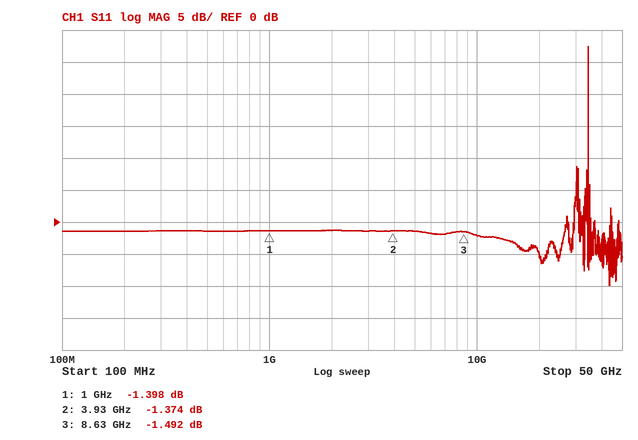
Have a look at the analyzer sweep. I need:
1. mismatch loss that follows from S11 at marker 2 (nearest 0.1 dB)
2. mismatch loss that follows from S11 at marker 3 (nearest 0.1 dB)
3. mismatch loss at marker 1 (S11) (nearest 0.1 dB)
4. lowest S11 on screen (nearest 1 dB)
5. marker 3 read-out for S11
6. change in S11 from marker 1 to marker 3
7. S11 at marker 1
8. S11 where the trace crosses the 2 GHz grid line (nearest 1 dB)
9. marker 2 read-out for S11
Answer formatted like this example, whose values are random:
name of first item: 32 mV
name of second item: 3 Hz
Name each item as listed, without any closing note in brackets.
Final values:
mismatch loss that follows from S11 at marker 2: 5.7 dB
mismatch loss that follows from S11 at marker 3: 5.4 dB
mismatch loss at marker 1 (S11): 5.6 dB
lowest S11 on screen: -10 dB
marker 3 read-out for S11: -1.492 dB
change in S11 from marker 1 to marker 3: -0.094 dB
S11 at marker 1: -1.398 dB
S11 where the trace crosses the 2 GHz grid line: -1 dB
marker 2 read-out for S11: -1.374 dB
